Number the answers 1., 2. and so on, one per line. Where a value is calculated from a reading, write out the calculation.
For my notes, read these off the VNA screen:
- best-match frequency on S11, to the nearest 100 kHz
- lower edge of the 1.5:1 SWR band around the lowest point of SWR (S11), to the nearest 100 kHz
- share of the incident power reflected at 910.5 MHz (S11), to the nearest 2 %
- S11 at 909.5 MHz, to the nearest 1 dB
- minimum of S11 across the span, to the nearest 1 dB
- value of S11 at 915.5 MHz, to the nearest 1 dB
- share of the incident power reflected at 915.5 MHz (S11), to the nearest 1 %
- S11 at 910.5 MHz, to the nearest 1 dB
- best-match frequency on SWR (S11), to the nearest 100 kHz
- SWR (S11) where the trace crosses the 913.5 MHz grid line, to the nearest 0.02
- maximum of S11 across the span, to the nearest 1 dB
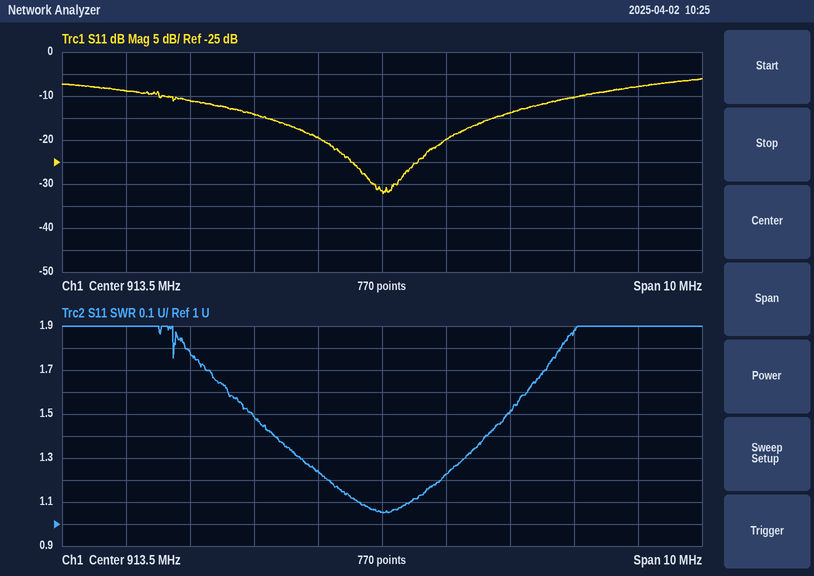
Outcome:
1. 913.5 MHz
2. 911.5 MHz
3. 10^(-11/10) ≈ 8 %
4. -9 dB
5. -32 dB
6. -14 dB
7. 10^(-14/10) ≈ 4 %
8. -11 dB
9. 913.5 MHz
10. 1.06
11. -6 dB
